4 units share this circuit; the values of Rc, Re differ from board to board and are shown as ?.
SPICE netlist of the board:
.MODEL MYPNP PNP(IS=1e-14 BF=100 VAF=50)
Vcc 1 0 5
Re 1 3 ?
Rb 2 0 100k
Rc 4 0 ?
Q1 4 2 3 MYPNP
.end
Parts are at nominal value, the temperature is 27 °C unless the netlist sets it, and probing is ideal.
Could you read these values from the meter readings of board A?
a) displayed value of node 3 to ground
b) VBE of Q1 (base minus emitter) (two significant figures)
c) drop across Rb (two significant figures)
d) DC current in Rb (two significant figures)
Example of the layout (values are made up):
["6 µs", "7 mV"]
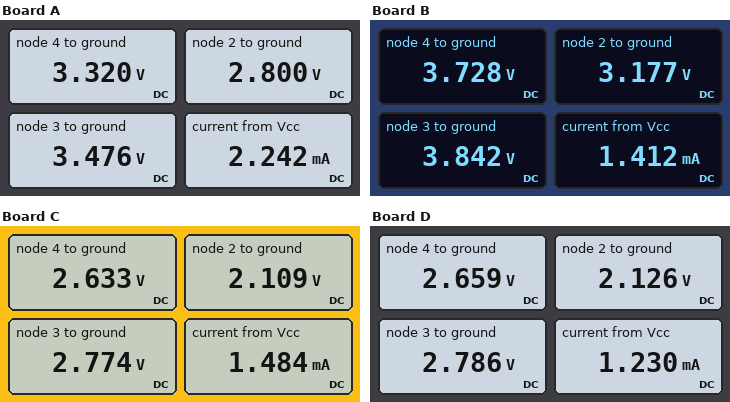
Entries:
["3.476 V", "-680 mV", "2.8 V", "28 µA"]
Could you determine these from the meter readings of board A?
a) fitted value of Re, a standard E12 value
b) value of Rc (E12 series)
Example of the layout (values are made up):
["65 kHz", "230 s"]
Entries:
["680 Ω", "1.5 kΩ"]
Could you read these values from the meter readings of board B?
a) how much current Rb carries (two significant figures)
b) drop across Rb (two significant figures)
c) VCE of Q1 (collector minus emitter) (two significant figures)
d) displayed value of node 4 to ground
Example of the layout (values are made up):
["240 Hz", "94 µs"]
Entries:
["32 µA", "3.2 V", "-110 mV", "3.728 V"]
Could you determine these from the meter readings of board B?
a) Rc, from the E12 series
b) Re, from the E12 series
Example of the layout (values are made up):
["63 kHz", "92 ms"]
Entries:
["2.7 kΩ", "820 Ω"]
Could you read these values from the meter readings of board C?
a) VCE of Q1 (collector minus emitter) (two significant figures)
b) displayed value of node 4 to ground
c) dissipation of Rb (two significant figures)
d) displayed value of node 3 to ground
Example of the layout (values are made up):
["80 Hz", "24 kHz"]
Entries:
["-140 mV", "2.633 V", "44 µW", "2.774 V"]
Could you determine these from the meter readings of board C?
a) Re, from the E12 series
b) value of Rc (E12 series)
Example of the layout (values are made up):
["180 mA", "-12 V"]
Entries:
["1.5 kΩ", "1.8 kΩ"]
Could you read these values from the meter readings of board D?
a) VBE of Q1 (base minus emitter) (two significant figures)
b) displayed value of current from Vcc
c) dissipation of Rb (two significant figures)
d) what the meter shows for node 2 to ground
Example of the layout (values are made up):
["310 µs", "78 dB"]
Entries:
["-660 mV", "1.230 mA", "45 µW", "2.126 V"]
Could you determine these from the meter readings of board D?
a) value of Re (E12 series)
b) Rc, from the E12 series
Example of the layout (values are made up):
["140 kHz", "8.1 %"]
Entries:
["1.8 kΩ", "2.2 kΩ"]
